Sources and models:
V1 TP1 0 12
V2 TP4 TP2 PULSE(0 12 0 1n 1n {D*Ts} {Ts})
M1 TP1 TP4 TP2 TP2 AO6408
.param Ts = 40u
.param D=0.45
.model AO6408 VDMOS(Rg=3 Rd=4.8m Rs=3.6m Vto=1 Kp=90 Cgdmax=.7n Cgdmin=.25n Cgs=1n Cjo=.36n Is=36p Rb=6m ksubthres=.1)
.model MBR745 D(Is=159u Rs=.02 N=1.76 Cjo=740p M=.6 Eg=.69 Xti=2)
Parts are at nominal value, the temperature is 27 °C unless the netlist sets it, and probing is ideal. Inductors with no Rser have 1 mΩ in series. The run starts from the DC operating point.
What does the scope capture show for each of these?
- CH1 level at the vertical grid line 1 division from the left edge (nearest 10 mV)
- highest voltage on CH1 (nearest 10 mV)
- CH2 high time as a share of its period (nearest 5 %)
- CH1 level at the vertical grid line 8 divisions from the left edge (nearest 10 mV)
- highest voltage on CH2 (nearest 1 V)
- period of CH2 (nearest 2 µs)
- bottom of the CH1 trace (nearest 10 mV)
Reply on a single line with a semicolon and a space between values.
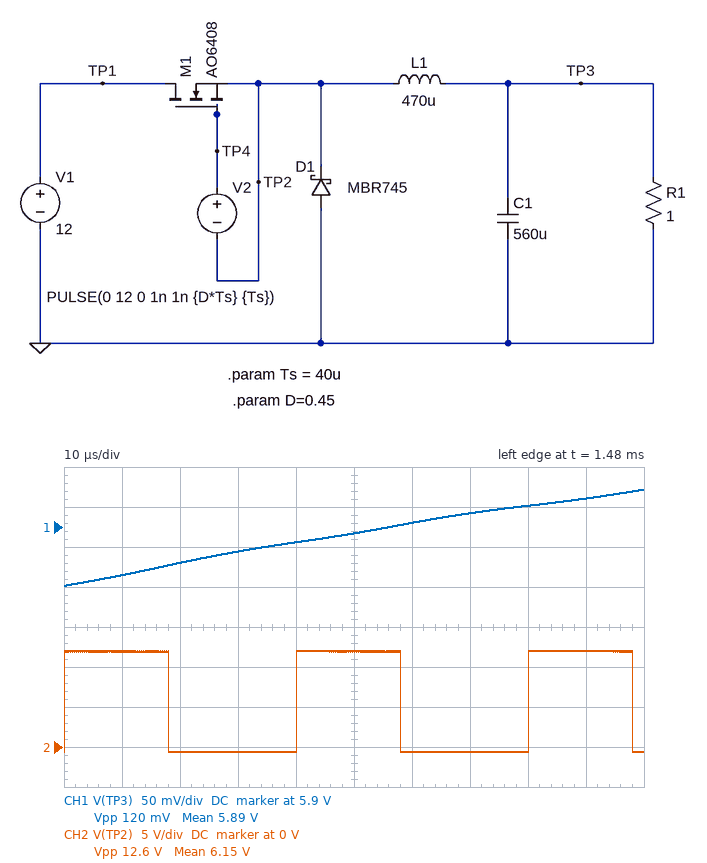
5.84 V; 5.95 V; 45 %; 5.93 V; 12 V; 40 µs; 5.83 V
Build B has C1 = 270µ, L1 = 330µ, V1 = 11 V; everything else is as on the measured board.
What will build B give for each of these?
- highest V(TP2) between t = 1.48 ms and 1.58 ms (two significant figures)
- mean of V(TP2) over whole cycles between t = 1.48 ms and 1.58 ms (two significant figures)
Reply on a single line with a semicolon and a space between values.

11 V; 4.6 V
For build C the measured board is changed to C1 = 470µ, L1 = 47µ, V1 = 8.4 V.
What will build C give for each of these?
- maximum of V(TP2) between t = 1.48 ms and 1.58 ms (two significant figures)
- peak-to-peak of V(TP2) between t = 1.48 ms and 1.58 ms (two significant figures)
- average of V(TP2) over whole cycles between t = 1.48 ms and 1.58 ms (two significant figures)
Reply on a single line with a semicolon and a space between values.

8.4 V; 8.9 V; 3.5 V
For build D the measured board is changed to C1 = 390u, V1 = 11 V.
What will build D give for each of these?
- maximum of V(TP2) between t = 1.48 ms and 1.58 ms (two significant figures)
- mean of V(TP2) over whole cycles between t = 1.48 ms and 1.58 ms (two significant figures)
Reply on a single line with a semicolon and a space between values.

11 V; 4.6 V
